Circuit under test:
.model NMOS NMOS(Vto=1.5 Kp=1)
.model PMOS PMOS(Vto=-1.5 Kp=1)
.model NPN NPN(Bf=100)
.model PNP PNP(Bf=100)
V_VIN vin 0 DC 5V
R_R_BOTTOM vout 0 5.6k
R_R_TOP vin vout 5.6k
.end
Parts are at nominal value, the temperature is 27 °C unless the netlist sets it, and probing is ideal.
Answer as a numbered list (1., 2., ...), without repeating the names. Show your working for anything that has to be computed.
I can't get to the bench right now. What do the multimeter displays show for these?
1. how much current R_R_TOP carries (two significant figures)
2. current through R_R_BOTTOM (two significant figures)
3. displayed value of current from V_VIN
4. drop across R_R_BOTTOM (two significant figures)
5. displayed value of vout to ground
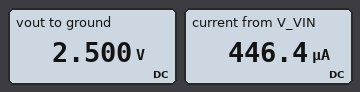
1. (5 V - 2.5 V) / 5.6 kΩ = 450 µA
2. (2.5 V) / 5.6 kΩ = 450 µA
3. 446.4 µA
4. 2.5 V = 2.5 V
5. 2.500 V
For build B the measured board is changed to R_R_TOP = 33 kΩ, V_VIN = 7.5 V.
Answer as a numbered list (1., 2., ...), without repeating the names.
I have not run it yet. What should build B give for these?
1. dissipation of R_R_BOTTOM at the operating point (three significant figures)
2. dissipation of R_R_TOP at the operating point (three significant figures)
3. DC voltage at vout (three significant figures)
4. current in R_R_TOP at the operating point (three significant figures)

1. 211 µW
2. 1.25 mW
3. 1.09 V
4. 194 µA
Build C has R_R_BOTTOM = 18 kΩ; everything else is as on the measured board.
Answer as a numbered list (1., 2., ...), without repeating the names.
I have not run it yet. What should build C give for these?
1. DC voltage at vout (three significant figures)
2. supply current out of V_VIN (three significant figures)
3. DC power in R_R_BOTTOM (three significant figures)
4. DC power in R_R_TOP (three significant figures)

1. 3.81 V
2. 212 µA
3. 808 µW
4. 251 µW
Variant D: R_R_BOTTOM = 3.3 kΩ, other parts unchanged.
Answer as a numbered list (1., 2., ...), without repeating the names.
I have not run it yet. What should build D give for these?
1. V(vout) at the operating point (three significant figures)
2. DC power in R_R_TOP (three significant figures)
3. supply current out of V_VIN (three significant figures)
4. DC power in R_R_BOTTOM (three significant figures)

1. 1.85 V
2. 1.77 mW
3. 562 µA
4. 1.04 mW
